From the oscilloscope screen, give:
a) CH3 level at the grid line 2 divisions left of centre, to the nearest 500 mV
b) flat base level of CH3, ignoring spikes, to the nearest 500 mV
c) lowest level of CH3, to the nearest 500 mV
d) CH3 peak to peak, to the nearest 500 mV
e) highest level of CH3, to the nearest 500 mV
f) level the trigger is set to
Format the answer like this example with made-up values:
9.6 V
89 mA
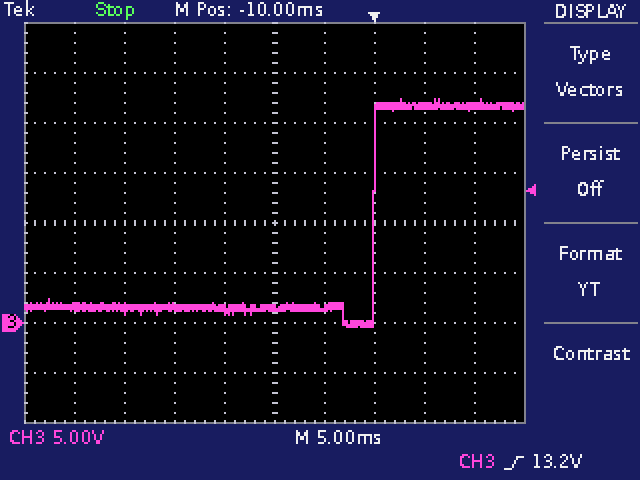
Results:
1.5 V
1.5 V
-500 mV
23.0 V
22.5 V
13.2 V
